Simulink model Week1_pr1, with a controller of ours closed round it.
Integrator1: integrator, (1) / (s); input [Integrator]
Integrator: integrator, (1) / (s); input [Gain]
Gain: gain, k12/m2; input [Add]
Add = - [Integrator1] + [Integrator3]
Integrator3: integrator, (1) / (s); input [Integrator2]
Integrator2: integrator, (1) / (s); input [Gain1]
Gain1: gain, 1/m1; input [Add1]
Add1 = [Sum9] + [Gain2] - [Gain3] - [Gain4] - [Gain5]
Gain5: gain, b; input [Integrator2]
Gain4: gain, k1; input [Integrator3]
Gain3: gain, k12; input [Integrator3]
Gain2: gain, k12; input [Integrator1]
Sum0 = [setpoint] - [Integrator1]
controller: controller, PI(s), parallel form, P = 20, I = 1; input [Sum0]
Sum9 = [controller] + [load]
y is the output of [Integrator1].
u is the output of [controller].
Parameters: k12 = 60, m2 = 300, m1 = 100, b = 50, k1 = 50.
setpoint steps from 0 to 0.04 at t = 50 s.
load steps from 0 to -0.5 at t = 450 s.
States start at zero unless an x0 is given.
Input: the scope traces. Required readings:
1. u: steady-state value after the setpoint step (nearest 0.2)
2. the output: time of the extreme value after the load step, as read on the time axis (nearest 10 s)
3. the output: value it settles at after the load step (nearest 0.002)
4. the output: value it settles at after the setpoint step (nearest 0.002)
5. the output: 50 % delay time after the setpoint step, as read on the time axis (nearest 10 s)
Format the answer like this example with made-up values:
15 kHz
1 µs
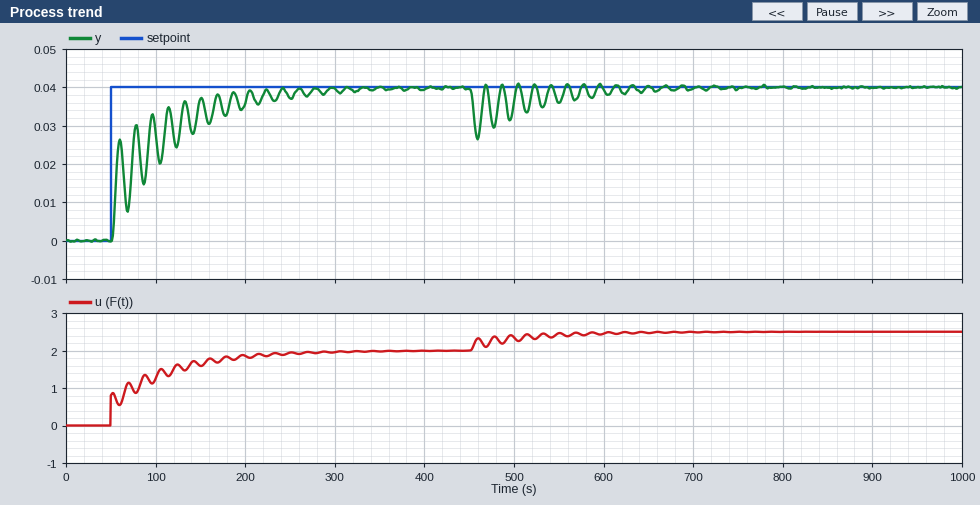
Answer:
2.0
460 s
0.040
0.040
60 s
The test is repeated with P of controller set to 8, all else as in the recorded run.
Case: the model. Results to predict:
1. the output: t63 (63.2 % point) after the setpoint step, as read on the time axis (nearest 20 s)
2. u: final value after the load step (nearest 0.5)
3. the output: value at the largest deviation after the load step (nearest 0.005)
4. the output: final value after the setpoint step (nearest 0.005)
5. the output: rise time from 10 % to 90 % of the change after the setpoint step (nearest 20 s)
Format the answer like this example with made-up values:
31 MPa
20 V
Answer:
100 s
2.5
0.025
0.040
100 s
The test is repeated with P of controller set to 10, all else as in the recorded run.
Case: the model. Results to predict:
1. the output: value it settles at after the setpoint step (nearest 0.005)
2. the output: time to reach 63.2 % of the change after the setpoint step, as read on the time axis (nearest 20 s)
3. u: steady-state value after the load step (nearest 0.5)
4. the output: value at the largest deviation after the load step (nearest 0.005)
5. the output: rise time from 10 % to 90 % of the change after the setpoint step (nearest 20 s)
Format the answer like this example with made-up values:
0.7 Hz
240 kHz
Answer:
0.040
100 s
2.5
0.025
100 s
